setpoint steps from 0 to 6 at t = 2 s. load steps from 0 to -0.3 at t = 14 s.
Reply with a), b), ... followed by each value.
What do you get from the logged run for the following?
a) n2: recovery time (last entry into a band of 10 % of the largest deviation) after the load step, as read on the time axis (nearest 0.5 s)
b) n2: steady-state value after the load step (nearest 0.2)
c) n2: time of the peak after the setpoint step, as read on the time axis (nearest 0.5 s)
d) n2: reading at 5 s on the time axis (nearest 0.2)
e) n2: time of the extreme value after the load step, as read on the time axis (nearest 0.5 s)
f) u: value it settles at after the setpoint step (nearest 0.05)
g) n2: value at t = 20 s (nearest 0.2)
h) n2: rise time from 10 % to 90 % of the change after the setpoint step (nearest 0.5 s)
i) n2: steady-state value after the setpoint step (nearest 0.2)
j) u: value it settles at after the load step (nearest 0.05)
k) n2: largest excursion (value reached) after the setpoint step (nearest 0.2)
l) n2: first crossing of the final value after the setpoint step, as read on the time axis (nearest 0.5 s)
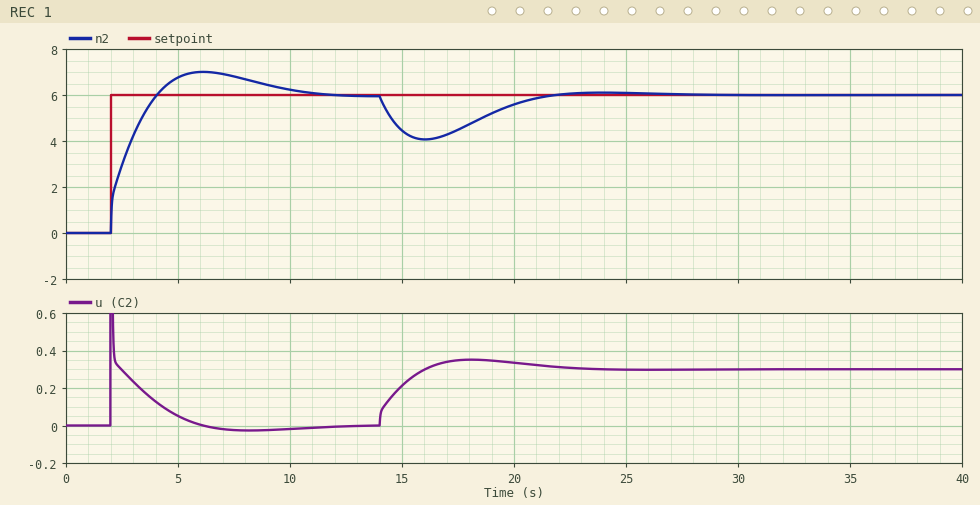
a) 21.0 s
b) 6.0
c) 6.0 s
d) 6.8
e) 16.0 s
f) 0.00
g) 5.6
h) 1.5 s
i) 6.0
j) 0.30
k) 7.0
l) 4.0 s
